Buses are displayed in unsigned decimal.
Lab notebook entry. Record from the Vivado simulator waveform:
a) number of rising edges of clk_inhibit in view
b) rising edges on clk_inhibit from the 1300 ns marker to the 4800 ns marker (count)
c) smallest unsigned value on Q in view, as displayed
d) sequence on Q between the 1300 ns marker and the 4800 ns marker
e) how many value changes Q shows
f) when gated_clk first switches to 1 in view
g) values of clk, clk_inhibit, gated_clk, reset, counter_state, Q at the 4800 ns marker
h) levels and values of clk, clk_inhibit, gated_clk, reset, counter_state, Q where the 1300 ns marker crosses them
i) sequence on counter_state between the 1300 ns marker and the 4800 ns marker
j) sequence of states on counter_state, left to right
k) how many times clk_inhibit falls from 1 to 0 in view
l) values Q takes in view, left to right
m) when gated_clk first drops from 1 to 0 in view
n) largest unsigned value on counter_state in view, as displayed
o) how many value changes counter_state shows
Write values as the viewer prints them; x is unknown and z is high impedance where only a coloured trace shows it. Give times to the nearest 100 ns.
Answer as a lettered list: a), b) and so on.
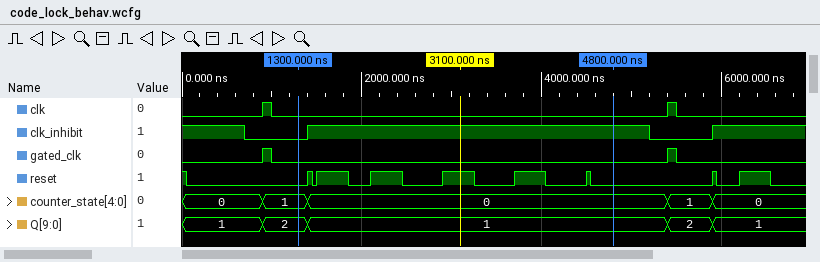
a) 2
b) 1
c) 1
d) 2, 1
e) 4
f) 900 ns
g) clk=0, clk_inhibit=1, gated_clk=0, reset=0, counter_state=0, Q=1
h) clk=0, clk_inhibit=0, gated_clk=0, reset=0, counter_state=1, Q=2
i) 1, 0
j) 0, 1, 0, 1, 0
k) 2
l) 1, 2, 1, 2, 1
m) 1000 ns
n) 1
o) 4
